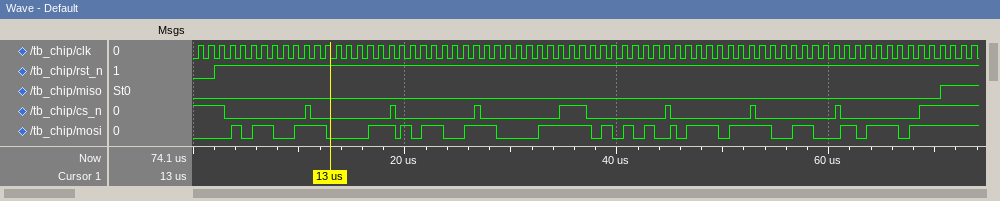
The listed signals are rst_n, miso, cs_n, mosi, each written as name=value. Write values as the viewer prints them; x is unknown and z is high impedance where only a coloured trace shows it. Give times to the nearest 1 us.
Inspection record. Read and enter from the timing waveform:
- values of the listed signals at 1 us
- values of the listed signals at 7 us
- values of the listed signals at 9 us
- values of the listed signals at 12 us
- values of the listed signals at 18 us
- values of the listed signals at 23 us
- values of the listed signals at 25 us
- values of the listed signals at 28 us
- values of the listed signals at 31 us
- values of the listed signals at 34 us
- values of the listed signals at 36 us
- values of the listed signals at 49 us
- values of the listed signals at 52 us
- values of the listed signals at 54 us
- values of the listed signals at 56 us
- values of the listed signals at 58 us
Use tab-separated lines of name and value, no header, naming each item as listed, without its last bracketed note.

values of the listed signals at 1 us	rst_n=0, miso=0, cs_n=1, mosi=0
values of the listed signals at 7 us	rst_n=1, miso=0, cs_n=0, mosi=1
values of the listed signals at 9 us	rst_n=1, miso=0, cs_n=0, mosi=0
values of the listed signals at 12 us	rst_n=1, miso=0, cs_n=0, mosi=1
values of the listed signals at 18 us	rst_n=1, miso=0, cs_n=0, mosi=1
values of the listed signals at 23 us	rst_n=1, miso=0, cs_n=0, mosi=1
values of the listed signals at 25 us	rst_n=1, miso=0, cs_n=0, mosi=0
values of the listed signals at 28 us	rst_n=1, miso=0, cs_n=0, mosi=1
values of the listed signals at 31 us	rst_n=1, miso=0, cs_n=0, mosi=0
values of the listed signals at 34 us	rst_n=1, miso=0, cs_n=0, mosi=1
values of the listed signals at 36 us	rst_n=1, miso=0, cs_n=1, mosi=1
values of the listed signals at 49 us	rst_n=1, miso=0, cs_n=0, mosi=1
values of the listed signals at 52 us	rst_n=1, miso=0, cs_n=0, mosi=1
values of the listed signals at 54 us	rst_n=1, miso=0, cs_n=0, mosi=1
values of the listed signals at 56 us	rst_n=1, miso=0, cs_n=0, mosi=0
values of the listed signals at 58 us	rst_n=1, miso=0, cs_n=0, mosi=1
